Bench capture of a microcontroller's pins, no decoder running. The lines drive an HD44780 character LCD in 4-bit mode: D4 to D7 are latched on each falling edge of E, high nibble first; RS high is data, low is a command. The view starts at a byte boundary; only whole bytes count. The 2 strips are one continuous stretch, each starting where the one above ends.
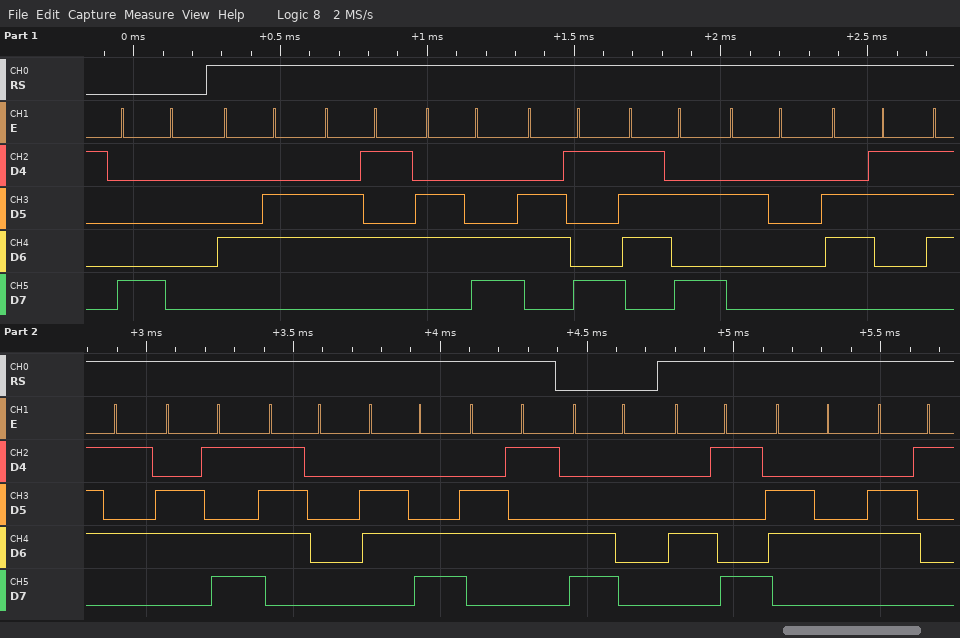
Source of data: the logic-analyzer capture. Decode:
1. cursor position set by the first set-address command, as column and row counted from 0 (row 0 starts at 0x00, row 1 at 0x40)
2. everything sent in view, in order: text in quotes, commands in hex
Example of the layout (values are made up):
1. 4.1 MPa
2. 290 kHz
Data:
1. column 0, row 0
2. 0x80 "Feliz cumple" 0xC0 "Ida"
